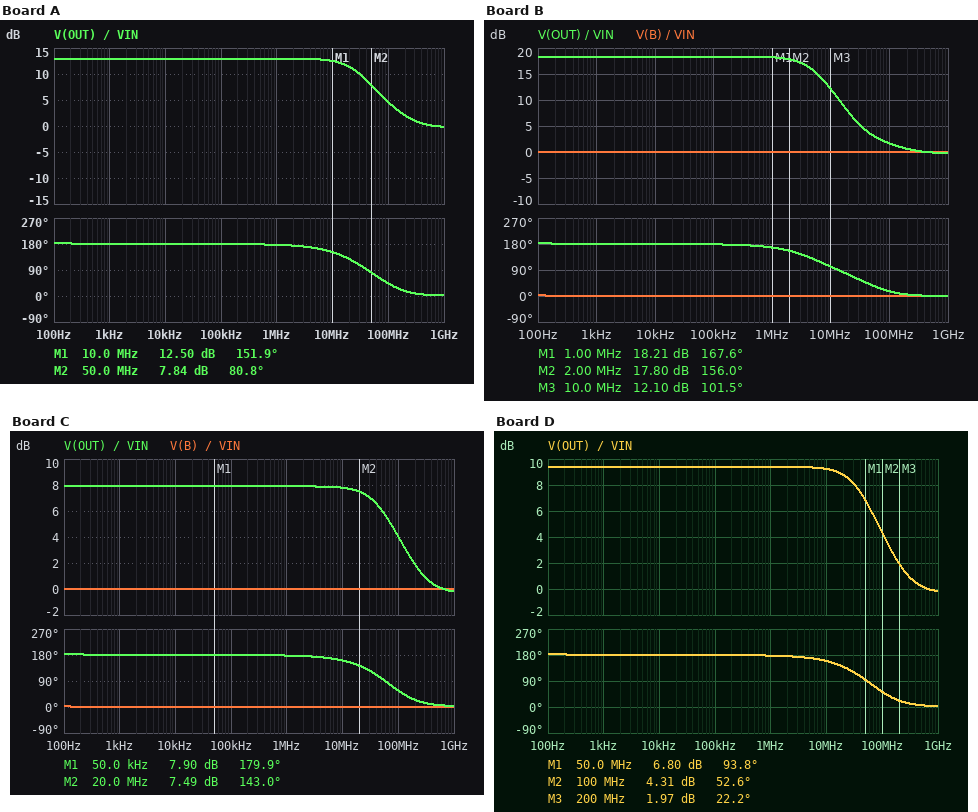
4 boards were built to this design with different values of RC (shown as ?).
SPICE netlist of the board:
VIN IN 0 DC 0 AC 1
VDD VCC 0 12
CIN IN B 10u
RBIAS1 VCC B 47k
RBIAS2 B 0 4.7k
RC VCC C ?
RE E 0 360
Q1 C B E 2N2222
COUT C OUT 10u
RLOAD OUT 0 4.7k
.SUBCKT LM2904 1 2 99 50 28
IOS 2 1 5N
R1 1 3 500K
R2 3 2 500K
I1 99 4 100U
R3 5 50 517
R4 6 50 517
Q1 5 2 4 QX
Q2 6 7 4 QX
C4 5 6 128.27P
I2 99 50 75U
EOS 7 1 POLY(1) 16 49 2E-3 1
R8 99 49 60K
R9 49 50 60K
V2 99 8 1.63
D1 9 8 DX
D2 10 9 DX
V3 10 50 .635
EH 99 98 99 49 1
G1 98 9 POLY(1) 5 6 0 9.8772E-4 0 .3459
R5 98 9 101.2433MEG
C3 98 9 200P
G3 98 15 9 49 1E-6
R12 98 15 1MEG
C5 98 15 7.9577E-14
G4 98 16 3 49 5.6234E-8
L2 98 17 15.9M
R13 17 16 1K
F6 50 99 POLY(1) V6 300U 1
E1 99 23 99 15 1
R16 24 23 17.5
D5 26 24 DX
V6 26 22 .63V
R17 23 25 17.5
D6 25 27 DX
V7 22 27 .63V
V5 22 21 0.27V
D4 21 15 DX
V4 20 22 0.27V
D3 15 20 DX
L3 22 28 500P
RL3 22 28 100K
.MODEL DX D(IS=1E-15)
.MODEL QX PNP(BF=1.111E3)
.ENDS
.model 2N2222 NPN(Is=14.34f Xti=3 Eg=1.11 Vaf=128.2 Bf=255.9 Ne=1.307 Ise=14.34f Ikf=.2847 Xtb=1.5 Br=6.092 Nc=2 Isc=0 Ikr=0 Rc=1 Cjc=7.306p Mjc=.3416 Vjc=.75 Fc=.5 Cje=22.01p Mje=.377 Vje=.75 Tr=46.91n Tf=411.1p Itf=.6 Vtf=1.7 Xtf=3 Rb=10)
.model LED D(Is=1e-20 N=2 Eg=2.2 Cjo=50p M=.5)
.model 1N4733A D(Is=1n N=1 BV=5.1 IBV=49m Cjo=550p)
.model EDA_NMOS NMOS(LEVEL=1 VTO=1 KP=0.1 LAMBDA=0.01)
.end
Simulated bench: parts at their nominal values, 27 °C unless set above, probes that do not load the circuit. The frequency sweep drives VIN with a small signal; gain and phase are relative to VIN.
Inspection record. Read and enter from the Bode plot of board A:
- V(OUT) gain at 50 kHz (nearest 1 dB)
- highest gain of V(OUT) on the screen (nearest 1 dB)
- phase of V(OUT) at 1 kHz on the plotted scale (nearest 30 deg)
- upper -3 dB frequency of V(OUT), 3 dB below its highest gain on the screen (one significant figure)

13 dB
13 dB
180 deg
30 MHz
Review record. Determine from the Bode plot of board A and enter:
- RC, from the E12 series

2.7 kΩ
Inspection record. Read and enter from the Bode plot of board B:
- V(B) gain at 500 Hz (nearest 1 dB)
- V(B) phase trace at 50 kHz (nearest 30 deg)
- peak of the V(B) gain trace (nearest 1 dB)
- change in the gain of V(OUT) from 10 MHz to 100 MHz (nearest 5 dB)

0 dB
0 deg
0 dB
-10 dB
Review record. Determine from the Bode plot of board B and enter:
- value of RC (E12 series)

10 kΩ
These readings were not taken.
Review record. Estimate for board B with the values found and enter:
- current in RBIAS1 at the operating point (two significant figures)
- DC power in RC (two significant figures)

230 µA
13 mW
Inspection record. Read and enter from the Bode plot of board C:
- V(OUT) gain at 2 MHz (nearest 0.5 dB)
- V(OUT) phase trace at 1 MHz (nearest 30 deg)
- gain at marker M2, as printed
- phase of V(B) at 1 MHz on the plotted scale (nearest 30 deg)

8.0 dB
180 deg
7.49 dB
0 deg
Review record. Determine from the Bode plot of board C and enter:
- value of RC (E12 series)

1.2 kΩ
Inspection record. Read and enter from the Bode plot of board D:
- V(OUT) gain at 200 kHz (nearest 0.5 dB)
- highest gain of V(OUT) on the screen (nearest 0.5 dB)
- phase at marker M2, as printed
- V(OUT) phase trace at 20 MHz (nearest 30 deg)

9.5 dB
9.5 dB
52.6 deg
150 deg
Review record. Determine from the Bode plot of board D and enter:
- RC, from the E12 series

1.5 kΩ
